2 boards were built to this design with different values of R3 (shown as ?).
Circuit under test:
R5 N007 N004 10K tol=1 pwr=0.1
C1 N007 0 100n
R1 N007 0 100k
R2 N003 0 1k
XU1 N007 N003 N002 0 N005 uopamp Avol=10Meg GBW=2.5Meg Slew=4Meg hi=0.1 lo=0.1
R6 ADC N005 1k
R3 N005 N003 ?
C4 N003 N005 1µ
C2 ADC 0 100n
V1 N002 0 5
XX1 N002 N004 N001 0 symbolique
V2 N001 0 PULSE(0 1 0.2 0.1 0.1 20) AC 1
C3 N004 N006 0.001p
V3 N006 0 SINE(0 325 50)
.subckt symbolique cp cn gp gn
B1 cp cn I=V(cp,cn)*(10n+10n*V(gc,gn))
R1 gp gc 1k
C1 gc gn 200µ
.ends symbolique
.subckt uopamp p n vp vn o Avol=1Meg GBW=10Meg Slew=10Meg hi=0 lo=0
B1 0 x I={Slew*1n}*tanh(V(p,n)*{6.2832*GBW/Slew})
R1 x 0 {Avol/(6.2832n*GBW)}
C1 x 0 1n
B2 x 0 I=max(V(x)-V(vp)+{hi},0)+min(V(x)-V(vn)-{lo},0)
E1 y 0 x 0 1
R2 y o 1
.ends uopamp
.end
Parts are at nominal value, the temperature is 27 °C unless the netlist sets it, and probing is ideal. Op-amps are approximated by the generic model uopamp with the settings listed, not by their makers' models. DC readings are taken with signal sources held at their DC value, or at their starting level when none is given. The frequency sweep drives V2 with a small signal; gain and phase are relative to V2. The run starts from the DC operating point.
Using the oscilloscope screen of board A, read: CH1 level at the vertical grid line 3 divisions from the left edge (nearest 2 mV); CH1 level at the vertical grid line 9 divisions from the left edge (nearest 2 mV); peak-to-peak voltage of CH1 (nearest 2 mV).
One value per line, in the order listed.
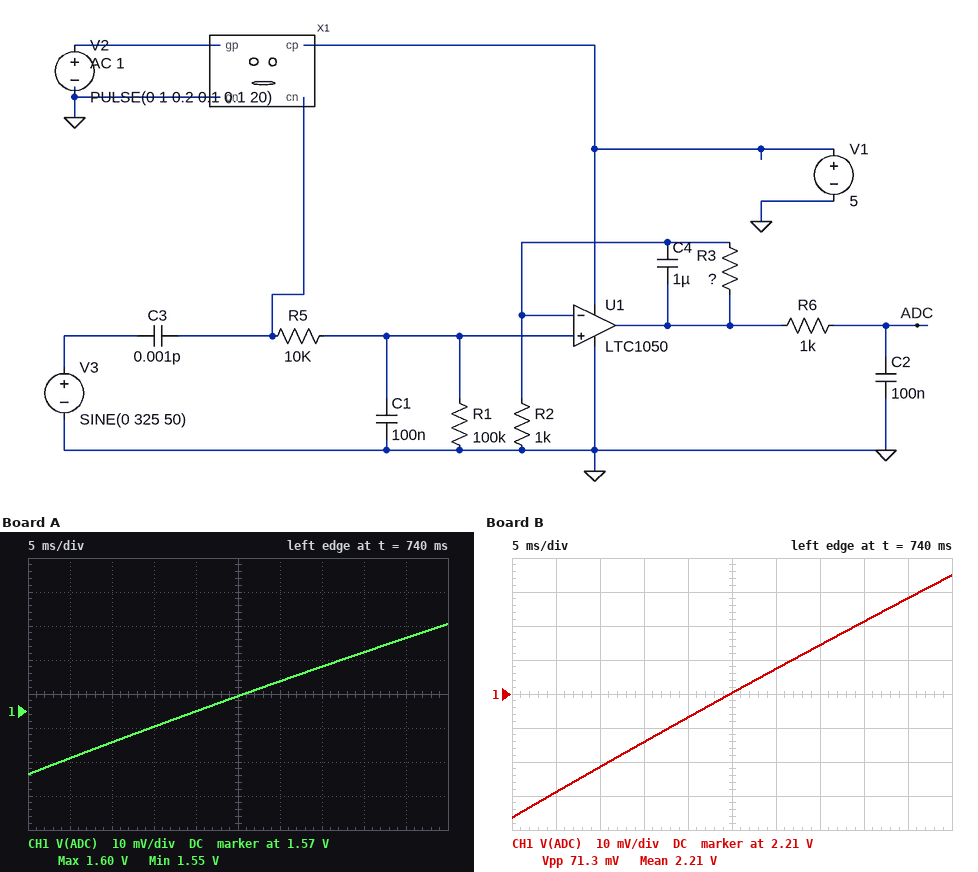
1.566 V
1.592 V
44 mV
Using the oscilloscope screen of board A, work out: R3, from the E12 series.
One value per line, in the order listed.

180 kΩ
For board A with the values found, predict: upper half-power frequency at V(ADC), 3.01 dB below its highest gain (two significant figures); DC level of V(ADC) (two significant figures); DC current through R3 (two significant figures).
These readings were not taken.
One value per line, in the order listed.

540 mHz
900 mV
5.0 µA
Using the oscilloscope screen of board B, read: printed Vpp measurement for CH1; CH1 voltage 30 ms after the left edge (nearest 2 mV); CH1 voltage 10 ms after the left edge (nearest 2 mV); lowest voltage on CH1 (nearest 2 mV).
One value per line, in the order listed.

71.3 mV
2.218 V
2.188 V
2.174 V
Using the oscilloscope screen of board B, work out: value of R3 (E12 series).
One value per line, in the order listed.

270 kΩ
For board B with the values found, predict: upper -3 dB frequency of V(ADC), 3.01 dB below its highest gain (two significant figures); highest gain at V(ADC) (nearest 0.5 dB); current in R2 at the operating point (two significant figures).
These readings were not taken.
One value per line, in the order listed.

430 mHz
2.5 dB
5.0 µA
